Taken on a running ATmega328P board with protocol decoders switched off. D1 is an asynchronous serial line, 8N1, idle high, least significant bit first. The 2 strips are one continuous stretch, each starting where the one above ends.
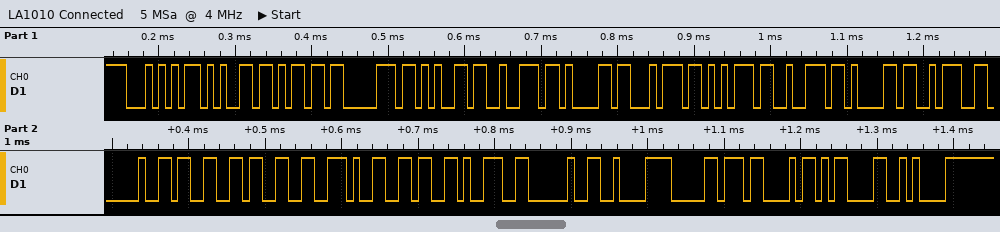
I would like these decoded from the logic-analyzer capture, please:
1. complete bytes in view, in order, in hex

54 65 6D 70 65 72 61 74 75 72 61 3A 20 33 33 2E 36 39 20 C2 B0 43 0D 0A
